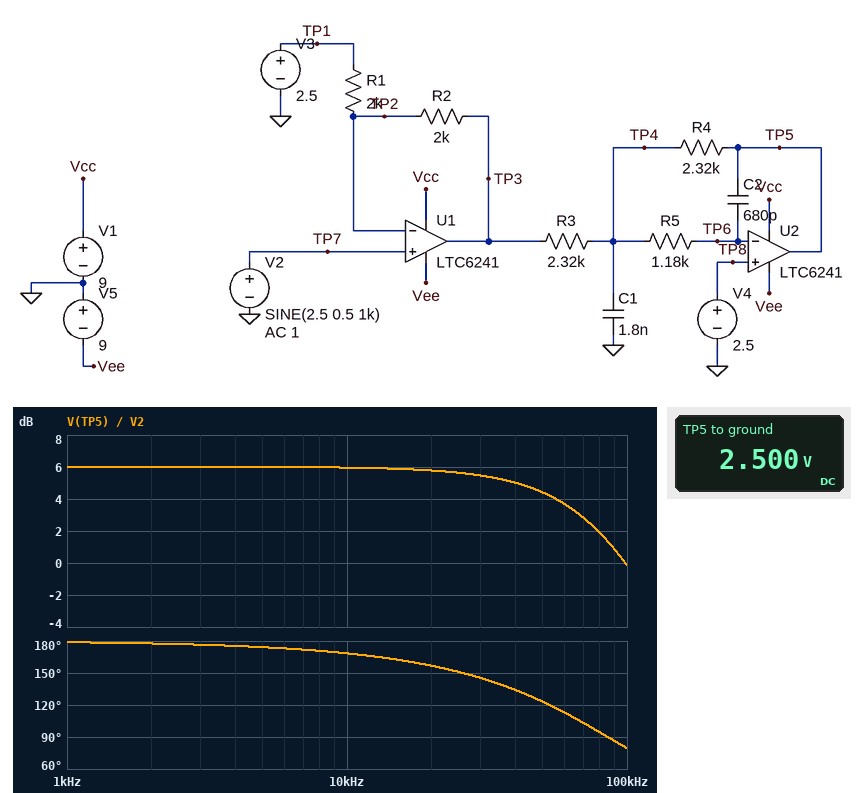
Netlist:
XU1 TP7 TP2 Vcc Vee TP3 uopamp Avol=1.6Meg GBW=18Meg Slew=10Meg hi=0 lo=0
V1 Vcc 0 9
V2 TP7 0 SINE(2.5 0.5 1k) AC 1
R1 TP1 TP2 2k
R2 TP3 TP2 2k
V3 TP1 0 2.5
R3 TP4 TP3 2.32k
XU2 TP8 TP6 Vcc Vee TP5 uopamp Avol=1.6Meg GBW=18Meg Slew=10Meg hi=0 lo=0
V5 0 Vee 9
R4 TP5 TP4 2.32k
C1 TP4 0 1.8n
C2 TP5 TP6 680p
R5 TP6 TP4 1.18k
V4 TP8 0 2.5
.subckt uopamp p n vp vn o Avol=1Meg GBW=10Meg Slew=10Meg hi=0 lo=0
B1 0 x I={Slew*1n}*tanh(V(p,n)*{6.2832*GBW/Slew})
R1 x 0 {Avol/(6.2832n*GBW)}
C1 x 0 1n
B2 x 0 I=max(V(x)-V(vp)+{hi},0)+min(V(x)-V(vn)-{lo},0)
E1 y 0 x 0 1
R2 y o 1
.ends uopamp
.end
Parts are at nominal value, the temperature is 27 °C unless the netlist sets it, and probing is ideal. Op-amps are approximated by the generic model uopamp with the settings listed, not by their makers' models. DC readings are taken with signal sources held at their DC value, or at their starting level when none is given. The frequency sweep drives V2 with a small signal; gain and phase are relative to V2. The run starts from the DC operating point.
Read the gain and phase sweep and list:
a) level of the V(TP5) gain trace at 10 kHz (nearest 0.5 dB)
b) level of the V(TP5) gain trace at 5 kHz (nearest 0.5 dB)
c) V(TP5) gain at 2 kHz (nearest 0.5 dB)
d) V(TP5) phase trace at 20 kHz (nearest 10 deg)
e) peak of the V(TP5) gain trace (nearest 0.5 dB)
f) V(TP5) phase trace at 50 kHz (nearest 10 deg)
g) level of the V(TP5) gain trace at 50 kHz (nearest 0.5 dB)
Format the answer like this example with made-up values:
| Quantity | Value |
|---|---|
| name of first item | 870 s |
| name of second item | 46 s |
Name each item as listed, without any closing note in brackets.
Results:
| Quantity | Value |
|---|---|
| level of the V(TP5) gain trace at 10 kHz | 6.0 dB |
| level of the V(TP5) gain trace at 5 kHz | 6.0 dB |
| V(TP5) gain at 2 kHz | 6.0 dB |
| V(TP5) phase trace at 20 kHz | 160 deg |
| peak of the V(TP5) gain trace | 6.0 dB |
| V(TP5) phase trace at 50 kHz | 120 deg |
| level of the V(TP5) gain trace at 50 kHz | 4.5 dB |
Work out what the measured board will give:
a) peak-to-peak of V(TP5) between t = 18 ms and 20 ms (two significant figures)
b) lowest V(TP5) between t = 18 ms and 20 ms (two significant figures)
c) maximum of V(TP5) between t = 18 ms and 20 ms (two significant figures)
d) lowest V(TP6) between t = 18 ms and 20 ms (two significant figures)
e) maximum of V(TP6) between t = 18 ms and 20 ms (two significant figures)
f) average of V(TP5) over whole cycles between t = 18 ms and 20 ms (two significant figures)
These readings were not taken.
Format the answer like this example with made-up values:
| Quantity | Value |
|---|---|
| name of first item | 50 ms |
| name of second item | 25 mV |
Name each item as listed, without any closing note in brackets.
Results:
| Quantity | Value |
|---|---|
| peak-to-peak of V(TP5) between t = 18 ms and 20 ms | 2.0 V |
| lowest V(TP5) between t = 18 ms and 20 ms | 1.5 V |
| maximum of V(TP5) between t = 18 ms and 20 ms | 3.5 V |
| lowest V(TP6) between t = 18 ms and 20 ms | 2.5 V |
| maximum of V(TP6) between t = 18 ms and 20 ms | 2.5 V |
| average of V(TP5) over whole cycles between t = 18 ms and 20 ms | 2.5 V |
